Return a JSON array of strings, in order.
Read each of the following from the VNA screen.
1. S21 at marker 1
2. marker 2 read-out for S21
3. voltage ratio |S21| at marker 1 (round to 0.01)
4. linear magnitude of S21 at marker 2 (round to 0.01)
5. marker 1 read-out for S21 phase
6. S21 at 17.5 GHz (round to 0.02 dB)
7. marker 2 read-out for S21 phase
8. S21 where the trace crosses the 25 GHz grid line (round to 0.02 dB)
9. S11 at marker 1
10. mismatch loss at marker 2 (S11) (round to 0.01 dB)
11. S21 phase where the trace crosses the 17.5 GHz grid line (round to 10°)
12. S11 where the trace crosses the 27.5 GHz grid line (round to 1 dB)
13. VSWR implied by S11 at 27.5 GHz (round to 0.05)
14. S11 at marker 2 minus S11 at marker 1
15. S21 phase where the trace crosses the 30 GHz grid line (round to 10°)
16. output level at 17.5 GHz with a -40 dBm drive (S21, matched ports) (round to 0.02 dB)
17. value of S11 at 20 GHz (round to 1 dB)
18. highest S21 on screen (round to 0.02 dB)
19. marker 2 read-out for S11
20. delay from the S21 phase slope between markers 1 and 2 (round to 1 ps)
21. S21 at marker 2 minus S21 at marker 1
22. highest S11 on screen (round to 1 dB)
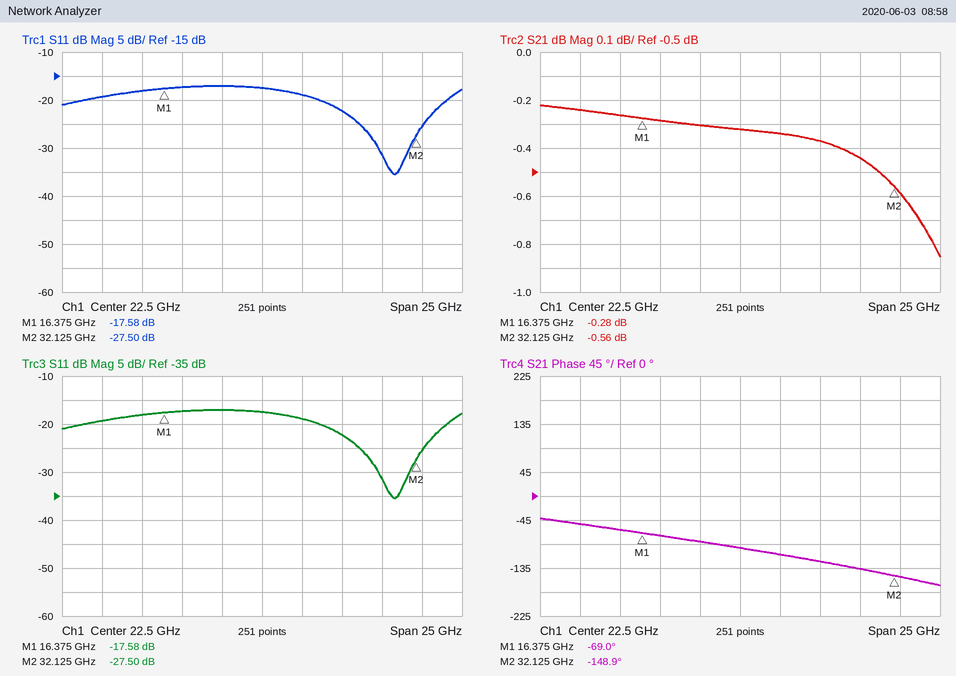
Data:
["-0.28 dB", "-0.56 dB", "0.97", "0.94", "-69.0°", "-0.28 dB", "-148.9°", "-0.34 dB", "-17.58 dB", "0.01 dB", "-70°", "-22 dB", "1.15", "-9.92 dB", "-140°", "-40.28 dBm", "-17 dB", "-0.22 dB", "-27.50 dB", "14 ps", "-0.28 dB", "-17 dB"]
